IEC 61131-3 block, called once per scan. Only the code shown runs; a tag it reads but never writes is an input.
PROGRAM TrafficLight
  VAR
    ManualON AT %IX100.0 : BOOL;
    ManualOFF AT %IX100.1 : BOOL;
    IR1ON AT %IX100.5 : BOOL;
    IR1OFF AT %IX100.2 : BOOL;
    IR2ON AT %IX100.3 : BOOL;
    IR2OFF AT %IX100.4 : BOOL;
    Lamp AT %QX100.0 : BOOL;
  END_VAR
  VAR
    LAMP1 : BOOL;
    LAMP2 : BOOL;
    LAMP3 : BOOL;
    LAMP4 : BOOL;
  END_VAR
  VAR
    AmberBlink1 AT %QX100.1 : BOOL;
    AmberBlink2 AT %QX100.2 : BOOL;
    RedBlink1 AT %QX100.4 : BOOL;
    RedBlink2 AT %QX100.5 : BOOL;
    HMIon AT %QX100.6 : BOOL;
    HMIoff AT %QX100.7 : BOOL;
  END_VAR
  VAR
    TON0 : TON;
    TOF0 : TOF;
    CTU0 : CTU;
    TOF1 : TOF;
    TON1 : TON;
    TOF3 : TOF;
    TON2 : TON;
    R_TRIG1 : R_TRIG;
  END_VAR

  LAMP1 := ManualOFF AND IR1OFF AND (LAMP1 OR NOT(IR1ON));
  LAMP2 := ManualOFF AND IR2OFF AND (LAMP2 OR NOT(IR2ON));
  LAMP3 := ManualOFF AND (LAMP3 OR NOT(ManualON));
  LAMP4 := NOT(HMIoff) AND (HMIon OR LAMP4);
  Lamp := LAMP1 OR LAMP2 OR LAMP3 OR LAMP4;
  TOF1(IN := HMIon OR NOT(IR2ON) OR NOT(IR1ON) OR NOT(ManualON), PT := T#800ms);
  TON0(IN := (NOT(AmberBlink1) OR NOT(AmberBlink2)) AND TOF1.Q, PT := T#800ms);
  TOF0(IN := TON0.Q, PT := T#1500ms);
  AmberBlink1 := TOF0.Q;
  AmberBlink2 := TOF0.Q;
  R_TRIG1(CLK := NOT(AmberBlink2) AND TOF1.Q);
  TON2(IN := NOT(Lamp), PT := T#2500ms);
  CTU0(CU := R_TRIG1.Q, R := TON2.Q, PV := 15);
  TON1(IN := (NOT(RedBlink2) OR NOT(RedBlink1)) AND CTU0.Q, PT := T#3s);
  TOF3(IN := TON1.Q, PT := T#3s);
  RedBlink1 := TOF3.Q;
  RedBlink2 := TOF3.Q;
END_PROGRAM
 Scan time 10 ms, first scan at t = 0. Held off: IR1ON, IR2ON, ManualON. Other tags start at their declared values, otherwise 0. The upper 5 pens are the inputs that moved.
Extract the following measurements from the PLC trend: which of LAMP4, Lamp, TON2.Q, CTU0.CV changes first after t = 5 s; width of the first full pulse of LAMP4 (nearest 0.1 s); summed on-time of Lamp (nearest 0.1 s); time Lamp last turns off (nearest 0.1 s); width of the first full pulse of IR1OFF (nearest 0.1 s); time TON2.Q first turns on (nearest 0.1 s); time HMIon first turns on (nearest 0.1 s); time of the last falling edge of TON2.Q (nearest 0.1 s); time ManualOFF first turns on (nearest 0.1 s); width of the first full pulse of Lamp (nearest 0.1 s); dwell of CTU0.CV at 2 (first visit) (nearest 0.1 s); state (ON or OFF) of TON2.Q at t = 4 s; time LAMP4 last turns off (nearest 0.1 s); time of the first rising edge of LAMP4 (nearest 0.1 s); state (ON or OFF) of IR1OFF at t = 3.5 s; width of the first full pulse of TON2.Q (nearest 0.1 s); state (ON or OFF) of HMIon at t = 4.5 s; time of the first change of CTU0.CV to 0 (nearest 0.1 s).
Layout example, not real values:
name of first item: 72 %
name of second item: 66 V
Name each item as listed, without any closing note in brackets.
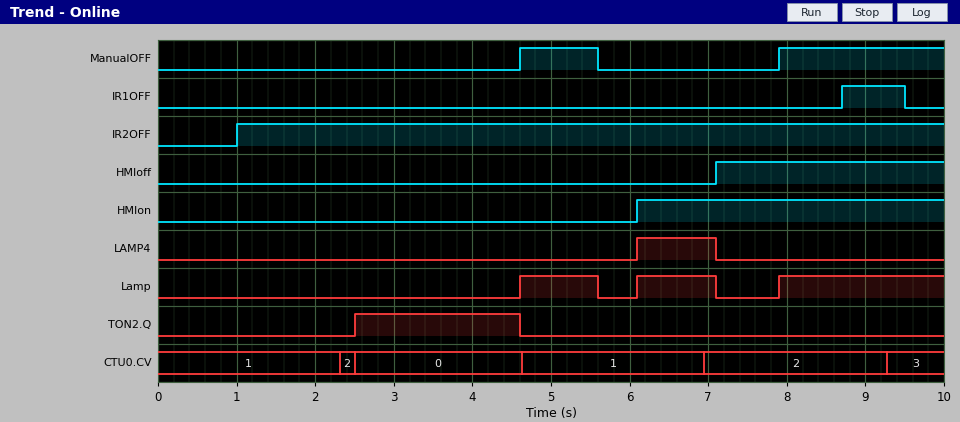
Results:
which of LAMP4, Lamp, TON2.Q, CTU0.CV changes first after t = 5 s: Lamp
width of the first full pulse of LAMP4: 1.0 s
summed on-time of Lamp: 4.1 s
time Lamp last turns off: 7.1 s
width of the first full pulse of IR1OFF: 0.8 s
time TON2.Q first turns on: 2.5 s
time HMIon first turns on: 6.1 s
time of the last falling edge of TON2.Q: 4.6 s
time ManualOFF first turns on: 4.6 s
width of the first full pulse of Lamp: 1.0 s
dwell of CTU0.CV at 2 (first visit): 0.2 s
state (ON or OFF) of TON2.Q at t = 4 s: ON
time LAMP4 last turns off: 7.1 s
time of the first rising edge of LAMP4: 6.1 s
state (ON or OFF) of IR1OFF at t = 3.5 s: OFF
width of the first full pulse of TON2.Q: 2.1 s
state (ON or OFF) of HMIon at t = 4.5 s: OFF
time of the first change of CTU0.CV to 0: 2.5 s
